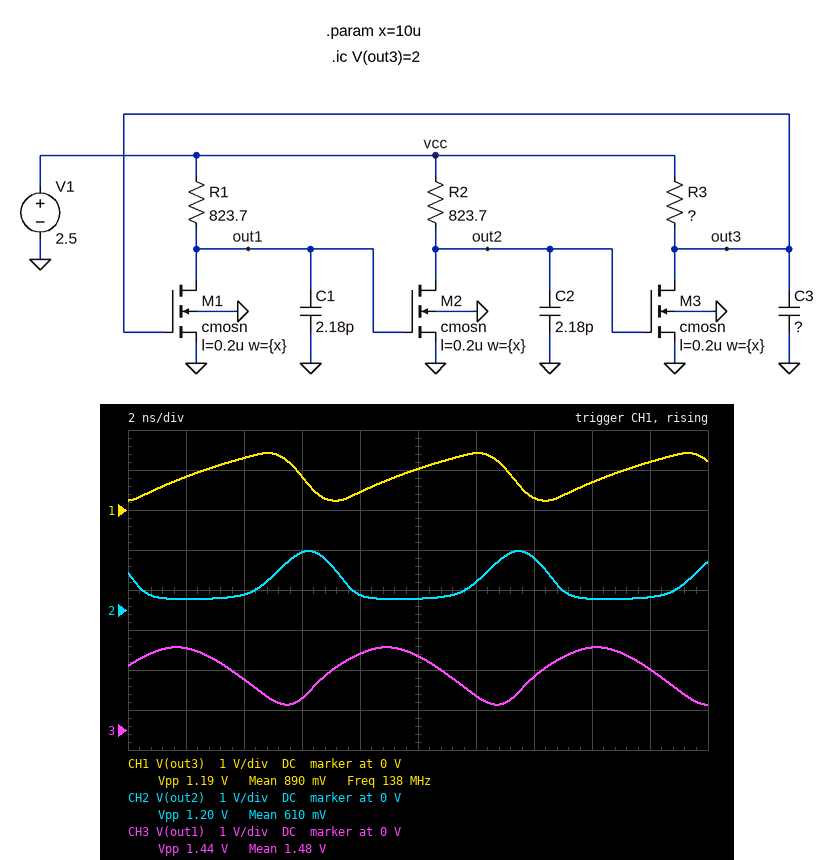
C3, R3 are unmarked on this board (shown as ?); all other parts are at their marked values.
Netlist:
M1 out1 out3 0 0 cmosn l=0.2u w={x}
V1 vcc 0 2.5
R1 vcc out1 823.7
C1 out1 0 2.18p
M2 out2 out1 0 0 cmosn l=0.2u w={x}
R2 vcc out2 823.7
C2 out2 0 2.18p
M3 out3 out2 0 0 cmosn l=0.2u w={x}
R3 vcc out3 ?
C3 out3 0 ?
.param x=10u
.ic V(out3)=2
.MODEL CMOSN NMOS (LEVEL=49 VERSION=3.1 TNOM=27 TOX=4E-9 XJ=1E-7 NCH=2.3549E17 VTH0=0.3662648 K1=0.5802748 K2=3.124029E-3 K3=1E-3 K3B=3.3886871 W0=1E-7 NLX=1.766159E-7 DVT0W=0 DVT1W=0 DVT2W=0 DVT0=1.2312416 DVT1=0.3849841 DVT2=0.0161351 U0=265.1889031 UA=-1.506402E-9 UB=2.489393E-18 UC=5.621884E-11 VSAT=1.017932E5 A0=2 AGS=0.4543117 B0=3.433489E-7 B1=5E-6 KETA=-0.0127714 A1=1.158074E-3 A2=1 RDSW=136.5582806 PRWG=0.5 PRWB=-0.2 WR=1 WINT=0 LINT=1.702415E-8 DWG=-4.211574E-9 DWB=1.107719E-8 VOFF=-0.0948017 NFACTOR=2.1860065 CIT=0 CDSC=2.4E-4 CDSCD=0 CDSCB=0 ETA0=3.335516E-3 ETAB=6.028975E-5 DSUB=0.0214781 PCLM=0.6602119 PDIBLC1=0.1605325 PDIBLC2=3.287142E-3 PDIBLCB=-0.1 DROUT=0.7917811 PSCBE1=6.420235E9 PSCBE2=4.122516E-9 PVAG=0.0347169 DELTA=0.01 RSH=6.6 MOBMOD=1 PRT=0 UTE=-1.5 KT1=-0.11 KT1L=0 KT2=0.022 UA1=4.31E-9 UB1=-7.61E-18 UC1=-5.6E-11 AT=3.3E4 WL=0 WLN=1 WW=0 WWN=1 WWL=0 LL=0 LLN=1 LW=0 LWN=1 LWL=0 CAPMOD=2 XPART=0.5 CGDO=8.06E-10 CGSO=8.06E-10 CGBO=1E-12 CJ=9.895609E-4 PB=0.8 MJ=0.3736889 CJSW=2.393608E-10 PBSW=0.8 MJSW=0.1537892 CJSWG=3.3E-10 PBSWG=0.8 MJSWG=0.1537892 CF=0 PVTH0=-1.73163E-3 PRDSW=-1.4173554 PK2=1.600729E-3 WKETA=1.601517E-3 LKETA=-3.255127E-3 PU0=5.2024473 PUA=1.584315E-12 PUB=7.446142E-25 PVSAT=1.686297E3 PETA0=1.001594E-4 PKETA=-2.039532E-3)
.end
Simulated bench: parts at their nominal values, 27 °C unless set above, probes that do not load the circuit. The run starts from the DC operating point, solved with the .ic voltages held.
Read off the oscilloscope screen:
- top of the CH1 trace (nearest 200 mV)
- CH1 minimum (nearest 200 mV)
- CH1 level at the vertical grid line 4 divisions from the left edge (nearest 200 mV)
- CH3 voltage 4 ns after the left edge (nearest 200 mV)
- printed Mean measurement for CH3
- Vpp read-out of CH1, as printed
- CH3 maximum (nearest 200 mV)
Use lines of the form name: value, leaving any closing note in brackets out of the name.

top of the CH1 trace: 1.4 V
CH1 minimum: 200 mV
CH1 level at the vertical grid line 4 divisions from the left edge: 400 mV
CH3 voltage 4 ns after the left edge: 1.2 V
printed Mean measurement for CH3: 1.48 V
Vpp read-out of CH1, as printed: 1.19 V
CH3 maximum: 2.0 V
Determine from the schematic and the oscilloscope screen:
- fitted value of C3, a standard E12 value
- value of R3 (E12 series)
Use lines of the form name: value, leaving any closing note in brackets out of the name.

fitted value of C3, a standard E12 value: 2.7 pF
value of R3: 2.2 kΩ
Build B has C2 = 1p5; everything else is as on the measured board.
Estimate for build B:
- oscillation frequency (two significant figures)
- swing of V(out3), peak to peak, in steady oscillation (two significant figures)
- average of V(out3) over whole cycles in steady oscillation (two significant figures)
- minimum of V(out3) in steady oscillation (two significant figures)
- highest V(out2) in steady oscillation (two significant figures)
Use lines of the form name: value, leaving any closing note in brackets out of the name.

oscillation frequency: 150 MHz
swing of V(out3), peak to peak, in steady oscillation: 1.1 V
average of V(out3) over whole cycles in steady oscillation: 880 mV
minimum of V(out3) in steady oscillation: 290 mV
highest V(out2) in steady oscillation: 1.5 V
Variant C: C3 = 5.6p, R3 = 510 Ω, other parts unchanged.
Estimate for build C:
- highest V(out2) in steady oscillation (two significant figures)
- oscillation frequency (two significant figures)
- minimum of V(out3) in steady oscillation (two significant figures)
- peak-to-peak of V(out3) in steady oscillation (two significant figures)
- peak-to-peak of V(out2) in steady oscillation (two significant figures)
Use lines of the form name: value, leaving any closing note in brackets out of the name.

highest V(out2) in steady oscillation: 2.0 V
oscillation frequency: 160 MHz
minimum of V(out3) in steady oscillation: 640 mV
peak-to-peak of V(out3) in steady oscillation: 1.0 V
peak-to-peak of V(out2) in steady oscillation: 1.6 V
